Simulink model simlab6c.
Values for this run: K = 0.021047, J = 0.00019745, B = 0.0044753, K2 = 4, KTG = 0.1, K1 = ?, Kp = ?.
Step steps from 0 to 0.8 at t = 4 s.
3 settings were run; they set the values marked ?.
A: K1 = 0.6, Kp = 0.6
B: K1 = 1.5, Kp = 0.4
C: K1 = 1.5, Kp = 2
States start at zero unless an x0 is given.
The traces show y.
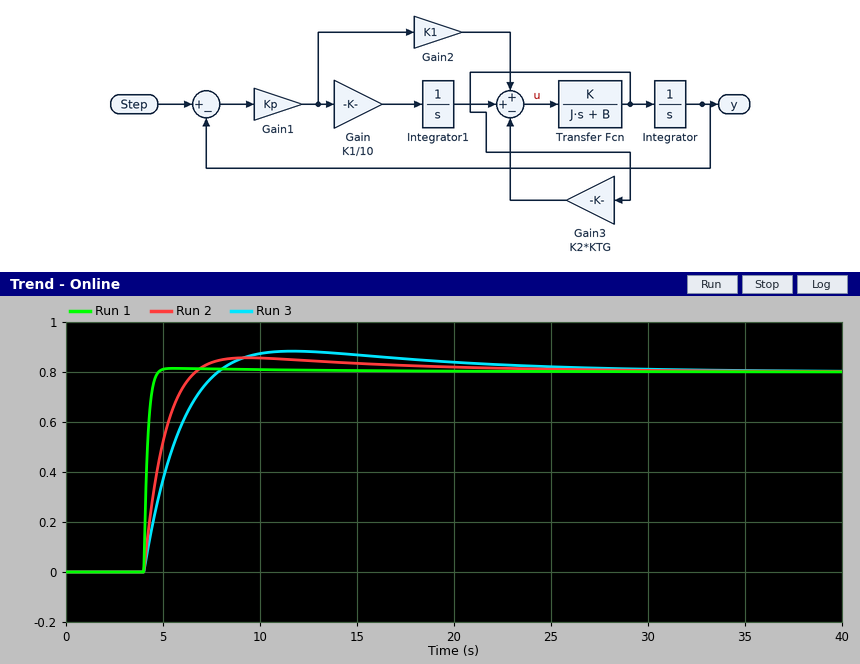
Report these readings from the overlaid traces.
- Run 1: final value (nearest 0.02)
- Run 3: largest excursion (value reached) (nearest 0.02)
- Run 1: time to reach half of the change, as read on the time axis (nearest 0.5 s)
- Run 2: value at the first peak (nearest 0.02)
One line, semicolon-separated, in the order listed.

0.80; 0.88; 4.0 s; 0.86
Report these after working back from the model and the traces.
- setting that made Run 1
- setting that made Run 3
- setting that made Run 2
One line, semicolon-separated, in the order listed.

C; A; B
